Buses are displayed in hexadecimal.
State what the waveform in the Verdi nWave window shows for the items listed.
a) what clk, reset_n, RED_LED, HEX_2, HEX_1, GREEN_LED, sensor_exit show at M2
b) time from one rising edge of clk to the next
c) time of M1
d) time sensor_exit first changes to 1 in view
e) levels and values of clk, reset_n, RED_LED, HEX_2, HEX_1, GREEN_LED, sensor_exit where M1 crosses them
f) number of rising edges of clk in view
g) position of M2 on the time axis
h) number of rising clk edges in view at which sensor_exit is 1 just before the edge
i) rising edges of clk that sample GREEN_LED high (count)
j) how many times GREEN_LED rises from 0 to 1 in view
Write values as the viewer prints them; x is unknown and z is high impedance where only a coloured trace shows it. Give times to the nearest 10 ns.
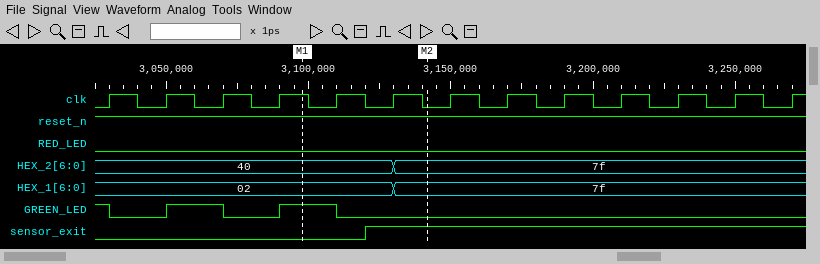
clk=0, reset_n=1, RED_LED=0, HEX_2=7f, HEX_1=7f, GREEN_LED=0, sensor_exit=1
20 ns
3100 ns
3120 ns
clk=1, reset_n=1, RED_LED=0, HEX_2=40, HEX_1=02, GREEN_LED=1, sensor_exit=0
13
3140 ns
8
3
2
